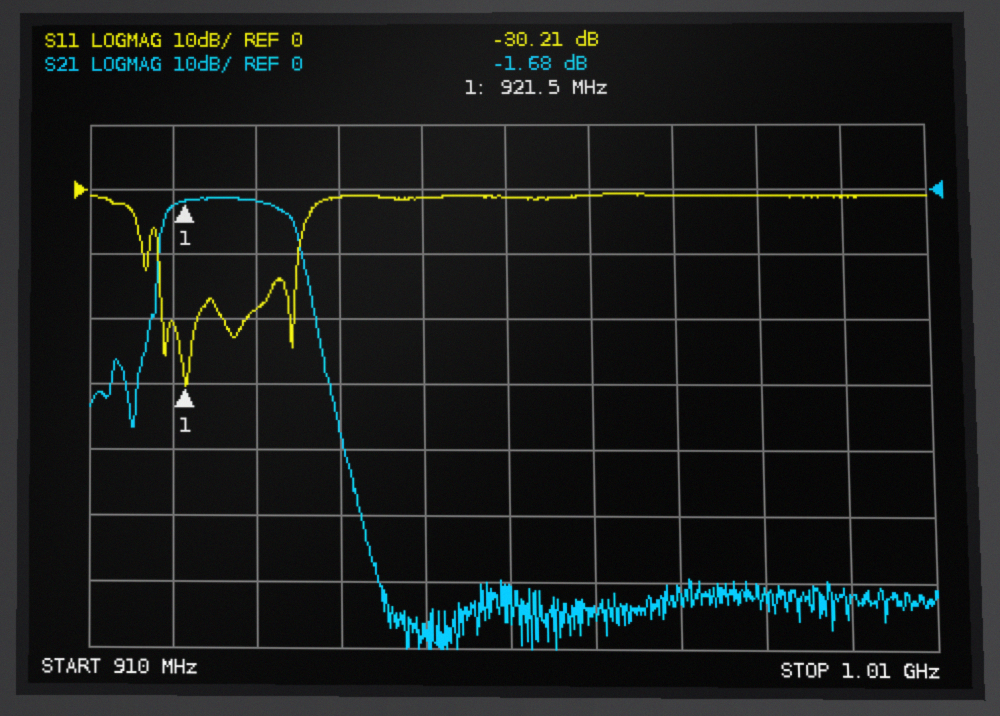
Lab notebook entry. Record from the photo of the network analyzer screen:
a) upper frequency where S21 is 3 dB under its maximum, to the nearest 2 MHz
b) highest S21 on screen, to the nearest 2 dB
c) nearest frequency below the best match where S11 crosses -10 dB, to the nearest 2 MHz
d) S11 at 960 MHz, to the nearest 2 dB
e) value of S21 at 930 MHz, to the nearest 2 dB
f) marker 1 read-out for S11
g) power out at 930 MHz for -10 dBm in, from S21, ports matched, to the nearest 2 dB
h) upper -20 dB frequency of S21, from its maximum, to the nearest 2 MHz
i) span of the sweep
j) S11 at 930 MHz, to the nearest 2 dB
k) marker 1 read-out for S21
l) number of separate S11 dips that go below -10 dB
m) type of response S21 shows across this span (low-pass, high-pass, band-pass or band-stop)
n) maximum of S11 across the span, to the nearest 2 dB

934 MHz
-2 dB
918 MHz
-2 dB
-2 dB
-30.21 dB
-12 dBm
938 MHz
100 MHz
-18 dB
-1.68 dB
5
band-pass
0 dB
